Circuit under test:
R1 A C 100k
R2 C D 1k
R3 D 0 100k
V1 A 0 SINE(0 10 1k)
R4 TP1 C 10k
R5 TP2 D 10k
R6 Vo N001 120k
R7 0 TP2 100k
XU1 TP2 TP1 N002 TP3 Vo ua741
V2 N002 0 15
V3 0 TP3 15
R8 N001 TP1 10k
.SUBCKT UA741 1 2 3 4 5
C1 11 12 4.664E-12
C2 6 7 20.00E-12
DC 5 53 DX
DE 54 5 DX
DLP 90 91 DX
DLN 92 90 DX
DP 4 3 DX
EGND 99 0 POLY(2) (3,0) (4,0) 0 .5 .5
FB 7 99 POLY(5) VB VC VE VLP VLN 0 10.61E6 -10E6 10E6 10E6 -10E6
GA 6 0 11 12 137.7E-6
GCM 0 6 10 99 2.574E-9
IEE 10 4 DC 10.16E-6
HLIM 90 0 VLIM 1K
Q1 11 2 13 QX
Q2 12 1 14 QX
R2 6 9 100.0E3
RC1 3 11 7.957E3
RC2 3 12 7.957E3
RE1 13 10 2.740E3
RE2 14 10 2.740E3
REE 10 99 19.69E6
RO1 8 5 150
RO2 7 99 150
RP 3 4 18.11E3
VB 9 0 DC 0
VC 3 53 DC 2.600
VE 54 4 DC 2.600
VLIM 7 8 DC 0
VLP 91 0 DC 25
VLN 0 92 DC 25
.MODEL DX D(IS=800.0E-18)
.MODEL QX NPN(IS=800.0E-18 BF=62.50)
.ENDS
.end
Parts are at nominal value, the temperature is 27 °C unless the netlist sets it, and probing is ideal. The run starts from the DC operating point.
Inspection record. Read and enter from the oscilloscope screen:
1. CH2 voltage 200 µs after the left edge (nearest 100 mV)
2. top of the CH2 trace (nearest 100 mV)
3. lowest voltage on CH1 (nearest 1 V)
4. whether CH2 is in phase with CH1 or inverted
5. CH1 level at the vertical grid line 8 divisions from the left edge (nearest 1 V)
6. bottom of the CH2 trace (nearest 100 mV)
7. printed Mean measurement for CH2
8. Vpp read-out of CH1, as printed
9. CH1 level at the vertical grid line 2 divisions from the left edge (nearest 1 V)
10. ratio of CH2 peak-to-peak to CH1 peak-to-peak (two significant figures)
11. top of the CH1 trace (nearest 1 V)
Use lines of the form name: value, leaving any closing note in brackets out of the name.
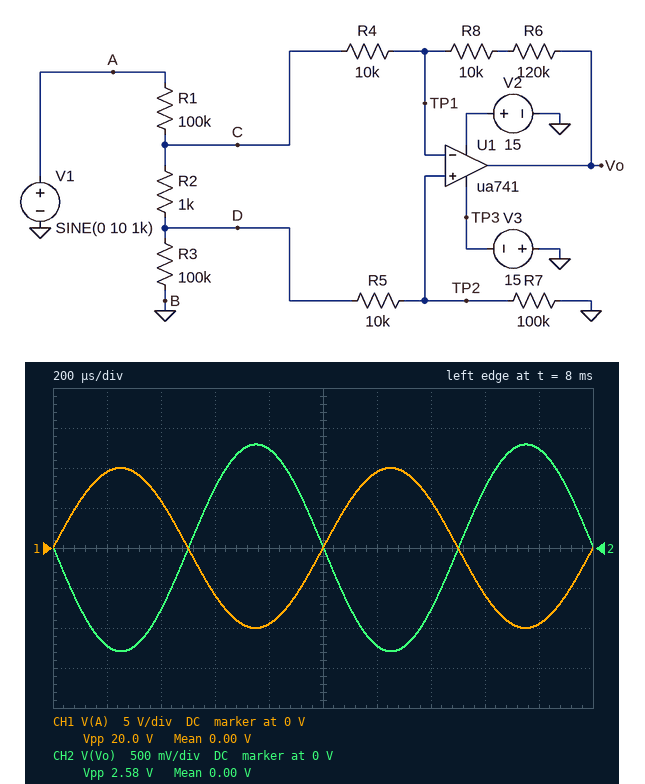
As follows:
CH2 voltage 200 µs after the left edge: -1.2 V
top of the CH2 trace: 1.3 V
lowest voltage on CH1: -10 V
whether CH2 is in phase with CH1 or inverted: inverted
CH1 level at the vertical grid line 8 divisions from the left edge: -6 V
bottom of the CH2 trace: -1.3 V
printed Mean measurement for CH2: 0.00 V
Vpp read-out of CH1, as printed: 20.0 V
CH1 level at the vertical grid line 2 divisions from the left edge: 6 V
ratio of CH2 peak-to-peak to CH1 peak-to-peak: 0.13
top of the CH1 trace: 10 V
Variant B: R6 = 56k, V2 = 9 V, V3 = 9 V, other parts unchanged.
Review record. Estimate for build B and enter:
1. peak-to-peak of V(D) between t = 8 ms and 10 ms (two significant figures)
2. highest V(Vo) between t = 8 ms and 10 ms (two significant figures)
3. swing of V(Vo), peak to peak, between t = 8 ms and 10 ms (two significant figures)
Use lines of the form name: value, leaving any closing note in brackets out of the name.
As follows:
peak-to-peak of V(D) between t = 8 ms and 10 ms: 5.0 V
highest V(Vo) between t = 8 ms and 10 ms: 450 mV
swing of V(Vo), peak to peak, between t = 8 ms and 10 ms: 910 mV
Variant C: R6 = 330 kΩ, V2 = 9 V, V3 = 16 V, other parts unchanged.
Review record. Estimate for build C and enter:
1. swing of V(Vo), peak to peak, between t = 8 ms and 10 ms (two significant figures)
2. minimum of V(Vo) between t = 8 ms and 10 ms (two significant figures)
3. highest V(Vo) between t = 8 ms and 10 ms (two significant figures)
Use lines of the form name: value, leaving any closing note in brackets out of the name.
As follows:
swing of V(Vo), peak to peak, between t = 8 ms and 10 ms: 14 V
minimum of V(Vo) between t = 8 ms and 10 ms: -7.0 V
highest V(Vo) between t = 8 ms and 10 ms: 6.9 V
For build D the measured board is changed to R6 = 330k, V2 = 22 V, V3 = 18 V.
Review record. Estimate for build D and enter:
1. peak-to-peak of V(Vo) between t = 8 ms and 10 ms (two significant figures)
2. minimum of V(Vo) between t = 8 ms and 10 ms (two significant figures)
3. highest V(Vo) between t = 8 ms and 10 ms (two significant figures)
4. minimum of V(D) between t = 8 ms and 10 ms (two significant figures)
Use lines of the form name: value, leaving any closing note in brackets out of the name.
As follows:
peak-to-peak of V(Vo) between t = 8 ms and 10 ms: 14 V
minimum of V(Vo) between t = 8 ms and 10 ms: -7.0 V
highest V(Vo) between t = 8 ms and 10 ms: 7.0 V
minimum of V(D) between t = 8 ms and 10 ms: -2.5 V
